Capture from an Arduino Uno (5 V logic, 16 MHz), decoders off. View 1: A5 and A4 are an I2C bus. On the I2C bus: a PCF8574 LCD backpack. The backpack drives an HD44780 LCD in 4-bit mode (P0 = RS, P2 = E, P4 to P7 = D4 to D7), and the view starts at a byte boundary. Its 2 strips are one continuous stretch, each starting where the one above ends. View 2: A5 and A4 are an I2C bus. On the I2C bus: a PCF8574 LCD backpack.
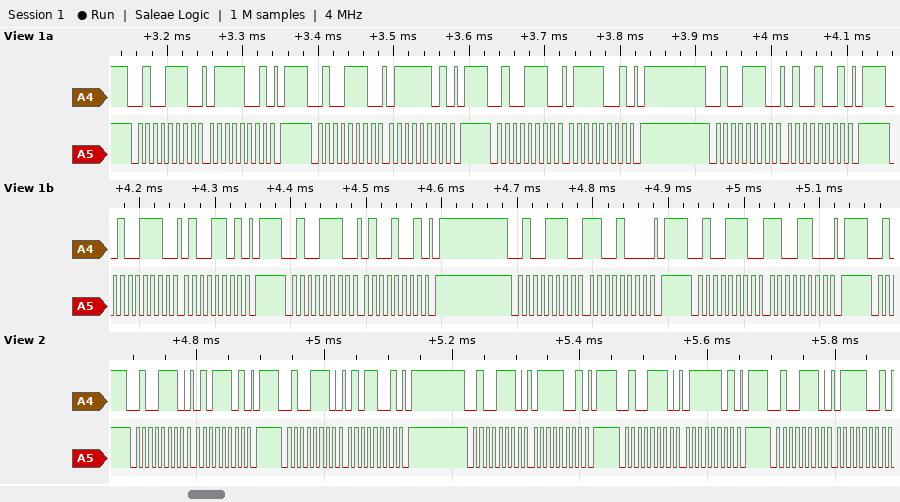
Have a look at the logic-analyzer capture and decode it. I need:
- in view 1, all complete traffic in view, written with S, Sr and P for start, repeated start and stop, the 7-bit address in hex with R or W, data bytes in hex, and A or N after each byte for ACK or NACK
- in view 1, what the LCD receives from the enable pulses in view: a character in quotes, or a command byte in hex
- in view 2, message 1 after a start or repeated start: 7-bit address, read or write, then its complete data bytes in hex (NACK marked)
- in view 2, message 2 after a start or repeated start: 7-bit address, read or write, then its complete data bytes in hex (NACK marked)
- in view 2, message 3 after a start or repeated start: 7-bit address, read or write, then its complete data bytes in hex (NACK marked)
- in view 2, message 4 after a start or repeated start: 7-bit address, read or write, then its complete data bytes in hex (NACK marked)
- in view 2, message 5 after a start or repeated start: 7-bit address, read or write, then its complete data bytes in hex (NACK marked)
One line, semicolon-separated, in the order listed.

S 27W A 79 A P S 27W A 7D A P S 27W A 79 A P S 27W A 49 A P S 27W A 4D A P S 27W A 49 A P S 27W A C8 A P S 27W A CC A P; 't'; 0x27 write: 5D; 0x27 write: 59; 0x27 write: 79; 0x27 write: 7D; 0x27 write: 79
